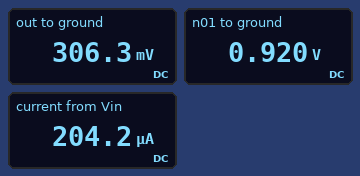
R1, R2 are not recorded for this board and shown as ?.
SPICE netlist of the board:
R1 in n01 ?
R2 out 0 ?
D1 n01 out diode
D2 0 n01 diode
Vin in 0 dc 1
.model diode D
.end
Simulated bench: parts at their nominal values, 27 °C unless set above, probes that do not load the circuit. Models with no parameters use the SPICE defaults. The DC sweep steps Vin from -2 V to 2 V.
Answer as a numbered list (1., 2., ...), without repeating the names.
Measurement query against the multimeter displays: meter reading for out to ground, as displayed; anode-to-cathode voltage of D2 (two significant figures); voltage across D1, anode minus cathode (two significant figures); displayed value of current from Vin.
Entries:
1. 306.3 mV
2. -920 mV
3. 610 mV
4. 204.2 µA
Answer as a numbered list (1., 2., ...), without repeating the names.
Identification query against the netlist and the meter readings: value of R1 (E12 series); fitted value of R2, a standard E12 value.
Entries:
1. 390 Ω
2. 1.5 kΩ
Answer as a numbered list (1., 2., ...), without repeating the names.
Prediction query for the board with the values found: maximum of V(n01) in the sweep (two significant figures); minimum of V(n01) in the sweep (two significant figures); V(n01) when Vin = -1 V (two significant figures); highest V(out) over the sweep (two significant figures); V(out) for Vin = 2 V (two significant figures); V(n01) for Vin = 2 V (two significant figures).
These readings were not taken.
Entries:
1. 1.7 V
2. -690 mV
3. -650 mV
4. 1.1 V
5. 1.1 V
6. 1.7 V
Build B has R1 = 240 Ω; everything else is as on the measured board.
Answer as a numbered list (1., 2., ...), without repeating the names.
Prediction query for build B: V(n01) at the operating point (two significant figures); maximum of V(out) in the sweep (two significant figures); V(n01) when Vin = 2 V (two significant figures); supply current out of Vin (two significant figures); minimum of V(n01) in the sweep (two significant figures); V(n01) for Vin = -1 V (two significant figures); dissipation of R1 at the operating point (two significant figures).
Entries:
1. 950 mV
2. 1.2 V
3. 1.8 V
4. 220 µA
5. -700 mV
6. -660 mV
7. 12 µW
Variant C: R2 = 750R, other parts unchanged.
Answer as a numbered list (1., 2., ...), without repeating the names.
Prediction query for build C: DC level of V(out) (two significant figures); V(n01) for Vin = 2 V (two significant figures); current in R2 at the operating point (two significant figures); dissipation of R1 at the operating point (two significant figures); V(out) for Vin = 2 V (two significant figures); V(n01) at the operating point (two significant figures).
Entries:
1. 250 mV
2. 1.5 V
3. 330 µA
4. 42 µW
5. 880 mV
6. 870 mV
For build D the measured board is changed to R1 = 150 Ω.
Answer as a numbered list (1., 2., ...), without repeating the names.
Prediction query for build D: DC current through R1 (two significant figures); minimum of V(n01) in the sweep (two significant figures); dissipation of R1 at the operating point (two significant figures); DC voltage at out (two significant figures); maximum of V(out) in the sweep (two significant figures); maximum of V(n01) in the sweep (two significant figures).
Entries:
1. 230 µA
2. -710 mV
3. 8.1 µW
4. 350 mV
5. 1.2 V
6. 1.9 V
